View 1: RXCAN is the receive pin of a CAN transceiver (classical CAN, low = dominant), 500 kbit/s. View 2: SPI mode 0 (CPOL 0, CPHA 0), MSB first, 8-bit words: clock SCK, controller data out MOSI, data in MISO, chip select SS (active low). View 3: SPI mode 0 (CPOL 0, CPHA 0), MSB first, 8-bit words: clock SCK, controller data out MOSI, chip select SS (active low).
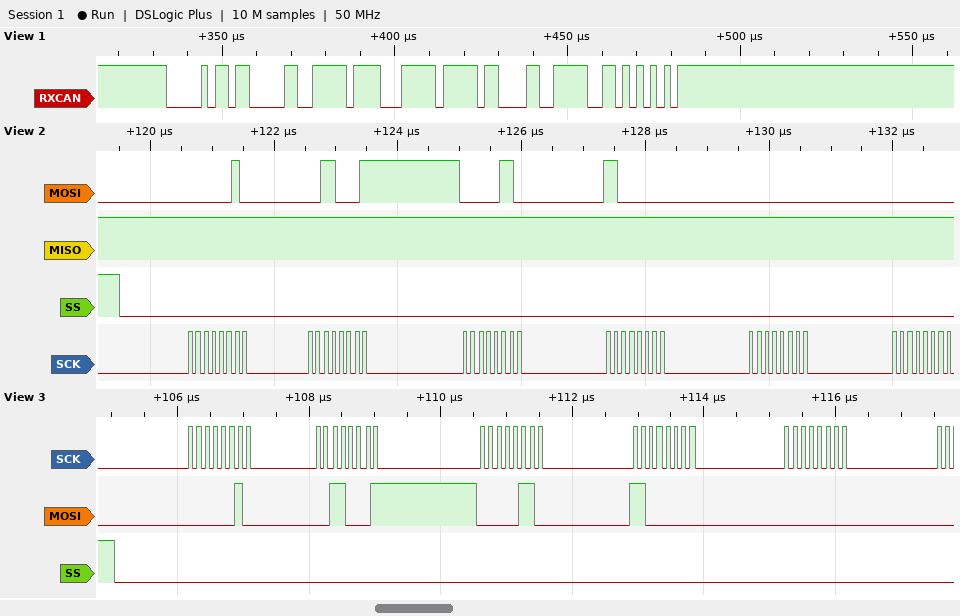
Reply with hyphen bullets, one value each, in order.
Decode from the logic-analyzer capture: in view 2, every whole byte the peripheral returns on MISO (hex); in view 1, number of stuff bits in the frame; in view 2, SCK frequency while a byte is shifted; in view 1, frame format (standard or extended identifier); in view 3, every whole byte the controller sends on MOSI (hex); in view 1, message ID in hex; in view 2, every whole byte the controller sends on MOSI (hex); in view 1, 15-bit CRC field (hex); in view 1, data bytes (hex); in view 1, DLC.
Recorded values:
- FF FF FF FF FF FF
- 6
- 8 MHz
- standard
- 02 31 06 C0 00
- 0x036
- 02 31 06 C0 00 00
- 0x7DAA
- FF 8F FF 0C
- 4
